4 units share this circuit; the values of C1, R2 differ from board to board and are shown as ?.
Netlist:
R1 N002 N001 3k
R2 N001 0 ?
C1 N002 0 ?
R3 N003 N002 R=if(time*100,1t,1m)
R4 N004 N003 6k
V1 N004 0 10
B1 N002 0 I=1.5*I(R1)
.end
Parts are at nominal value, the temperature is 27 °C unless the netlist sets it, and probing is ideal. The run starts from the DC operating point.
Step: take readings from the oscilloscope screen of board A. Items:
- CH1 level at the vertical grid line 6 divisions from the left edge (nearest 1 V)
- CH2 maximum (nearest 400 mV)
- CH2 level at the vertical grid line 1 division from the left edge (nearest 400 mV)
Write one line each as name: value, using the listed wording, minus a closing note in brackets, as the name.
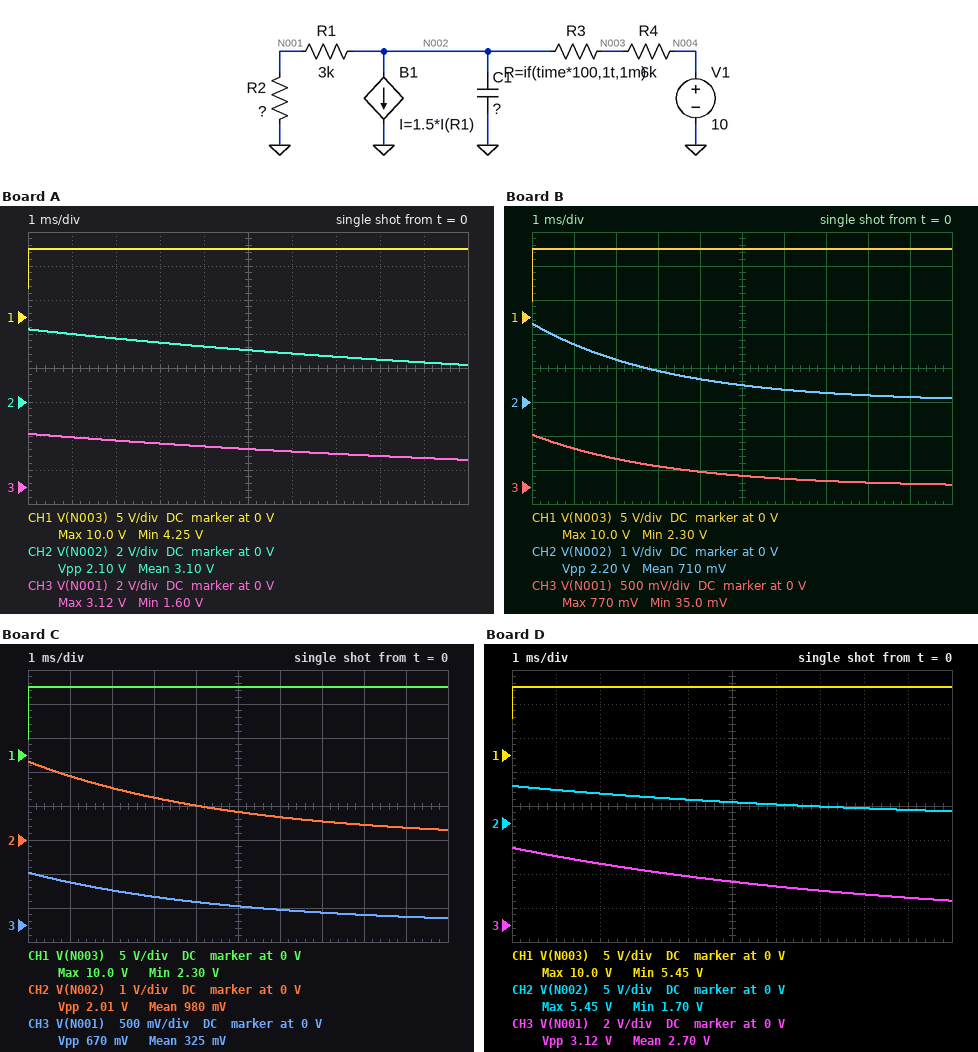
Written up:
CH1 level at the vertical grid line 6 divisions from the left edge: 10 V
CH2 maximum: 4.4 V
CH2 level at the vertical grid line 1 division from the left edge: 4.0 V
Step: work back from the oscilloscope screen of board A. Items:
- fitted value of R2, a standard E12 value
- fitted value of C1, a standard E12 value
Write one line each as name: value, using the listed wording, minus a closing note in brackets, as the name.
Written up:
fitted value of R2, a standard E12 value: 8.2 kΩ
fitted value of C1, a standard E12 value: 3.3 µF
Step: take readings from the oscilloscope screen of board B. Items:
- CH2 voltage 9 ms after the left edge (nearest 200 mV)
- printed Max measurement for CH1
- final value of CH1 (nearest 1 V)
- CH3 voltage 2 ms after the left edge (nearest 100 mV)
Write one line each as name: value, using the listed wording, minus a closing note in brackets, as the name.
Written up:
CH2 voltage 9 ms after the left edge: 200 mV
printed Max measurement for CH1: 10.0 V
final value of CH1: 10 V
CH3 voltage 2 ms after the left edge: 400 mV
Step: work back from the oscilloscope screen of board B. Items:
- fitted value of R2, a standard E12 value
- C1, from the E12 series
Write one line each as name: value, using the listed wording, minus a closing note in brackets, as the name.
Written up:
fitted value of R2, a standard E12 value: 1.5 kΩ
C1, from the E12 series: 1.8 µF
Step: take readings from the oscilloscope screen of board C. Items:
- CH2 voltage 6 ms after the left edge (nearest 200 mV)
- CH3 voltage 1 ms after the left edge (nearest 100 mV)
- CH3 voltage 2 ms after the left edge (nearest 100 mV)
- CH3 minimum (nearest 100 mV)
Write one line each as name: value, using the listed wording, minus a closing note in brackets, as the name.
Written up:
CH2 voltage 6 ms after the left edge: 600 mV
CH3 voltage 1 ms after the left edge: 600 mV
CH3 voltage 2 ms after the left edge: 500 mV
CH3 minimum: 100 mV
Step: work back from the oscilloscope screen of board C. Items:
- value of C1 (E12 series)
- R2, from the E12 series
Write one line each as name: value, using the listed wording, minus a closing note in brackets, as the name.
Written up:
value of C1: 2.7 µF
R2, from the E12 series: 1.5 kΩ
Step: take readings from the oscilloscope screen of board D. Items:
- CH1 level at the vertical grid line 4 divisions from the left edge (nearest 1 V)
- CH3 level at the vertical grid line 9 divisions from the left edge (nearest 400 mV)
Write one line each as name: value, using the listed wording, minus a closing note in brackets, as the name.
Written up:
CH1 level at the vertical grid line 4 divisions from the left edge: 10 V
CH3 level at the vertical grid line 9 divisions from the left edge: 1.6 V
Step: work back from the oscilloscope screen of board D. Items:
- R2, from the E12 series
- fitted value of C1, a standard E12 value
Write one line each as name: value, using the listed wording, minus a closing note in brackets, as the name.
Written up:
R2, from the E12 series: 15 kΩ
fitted value of C1, a standard E12 value: 1.2 µF
